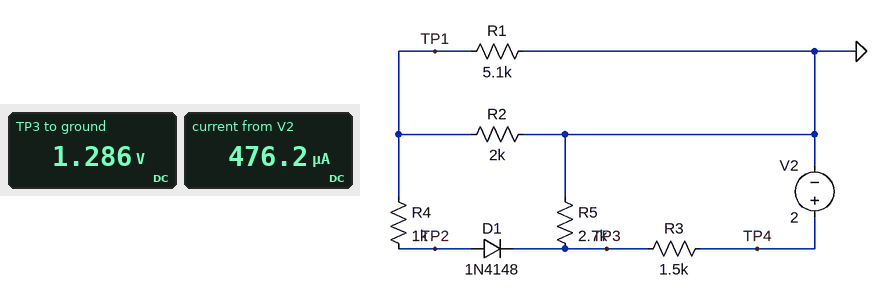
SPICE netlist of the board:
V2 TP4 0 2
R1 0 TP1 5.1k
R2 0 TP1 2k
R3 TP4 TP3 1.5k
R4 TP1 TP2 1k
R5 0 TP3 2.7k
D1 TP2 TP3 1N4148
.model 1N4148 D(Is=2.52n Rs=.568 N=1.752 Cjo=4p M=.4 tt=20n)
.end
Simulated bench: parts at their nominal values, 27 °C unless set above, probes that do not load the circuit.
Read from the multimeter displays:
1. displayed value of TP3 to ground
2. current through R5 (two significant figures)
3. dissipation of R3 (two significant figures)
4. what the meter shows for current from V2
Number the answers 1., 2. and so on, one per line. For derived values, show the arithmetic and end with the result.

1. 1.286 V
2. (1.286 V) / 2.7 kΩ = 480 µA
3. (2 V - 1.286 V)^2 / 1.5 kΩ = 340 µW
4. 476.2 µA
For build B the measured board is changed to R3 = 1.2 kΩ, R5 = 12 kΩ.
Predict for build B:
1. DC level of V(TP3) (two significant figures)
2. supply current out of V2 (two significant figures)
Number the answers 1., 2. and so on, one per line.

1. 1.8 V
2. 150 µA
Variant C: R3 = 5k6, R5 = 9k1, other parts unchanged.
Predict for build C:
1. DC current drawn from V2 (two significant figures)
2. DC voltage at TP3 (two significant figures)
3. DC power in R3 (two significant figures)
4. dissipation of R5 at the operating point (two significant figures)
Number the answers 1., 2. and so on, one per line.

1. 140 µA
2. 1.2 V
3. 100 µW
4. 170 µW
